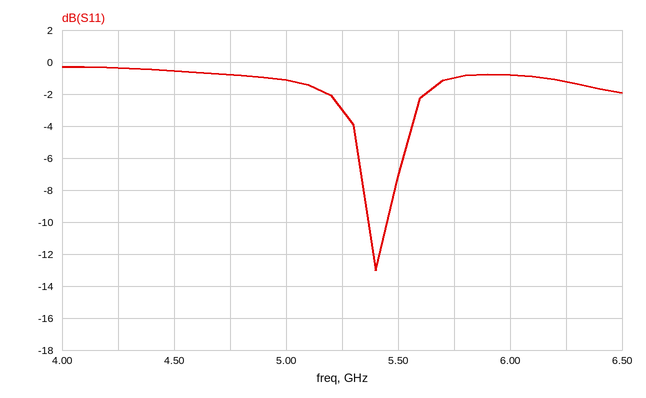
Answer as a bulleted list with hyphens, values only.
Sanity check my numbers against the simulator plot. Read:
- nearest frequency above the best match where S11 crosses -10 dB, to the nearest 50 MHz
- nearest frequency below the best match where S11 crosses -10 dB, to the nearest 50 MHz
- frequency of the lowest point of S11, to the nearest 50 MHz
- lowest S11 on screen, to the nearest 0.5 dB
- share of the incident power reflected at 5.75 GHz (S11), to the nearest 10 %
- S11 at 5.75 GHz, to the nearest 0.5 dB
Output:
- 5.45 GHz
- 5.35 GHz
- 5.40 GHz
- -13.0 dB
- 80 %
- -1.0 dB
